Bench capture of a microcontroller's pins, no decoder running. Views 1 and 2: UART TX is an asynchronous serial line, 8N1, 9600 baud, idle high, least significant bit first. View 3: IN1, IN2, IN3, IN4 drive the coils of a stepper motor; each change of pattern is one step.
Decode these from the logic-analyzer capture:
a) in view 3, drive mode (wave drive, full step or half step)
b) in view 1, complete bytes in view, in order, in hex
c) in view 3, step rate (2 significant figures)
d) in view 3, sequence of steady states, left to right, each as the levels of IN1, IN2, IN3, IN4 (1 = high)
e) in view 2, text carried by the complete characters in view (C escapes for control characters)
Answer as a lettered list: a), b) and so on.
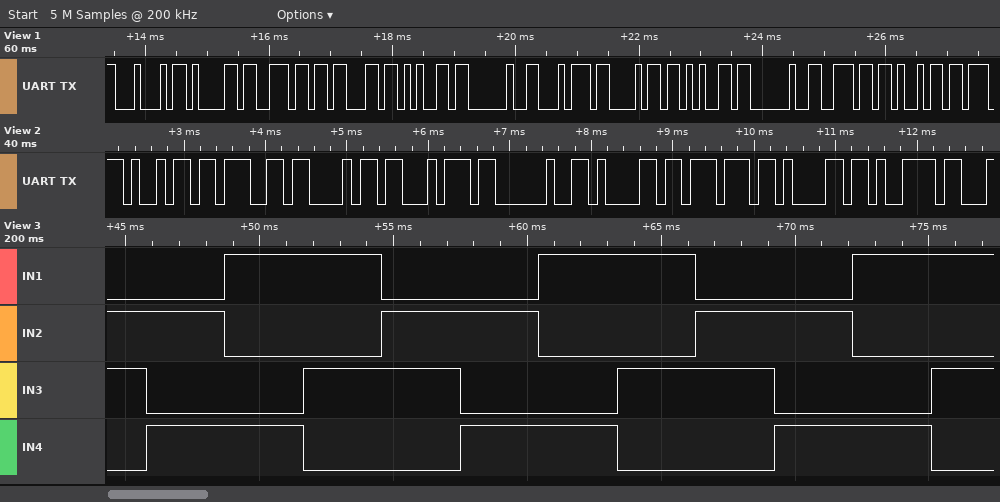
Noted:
a) full step
b) 0x44 0x61 0x6E 0x63 0x65 0x20 0x74 0x68 0x65 0x20 0x6E 0x69
c) 340 steps/s
d) 0110 0101 1001 1010 0110 0101 1001 1010 0110 0101 1001 1010
e) "ight away"
